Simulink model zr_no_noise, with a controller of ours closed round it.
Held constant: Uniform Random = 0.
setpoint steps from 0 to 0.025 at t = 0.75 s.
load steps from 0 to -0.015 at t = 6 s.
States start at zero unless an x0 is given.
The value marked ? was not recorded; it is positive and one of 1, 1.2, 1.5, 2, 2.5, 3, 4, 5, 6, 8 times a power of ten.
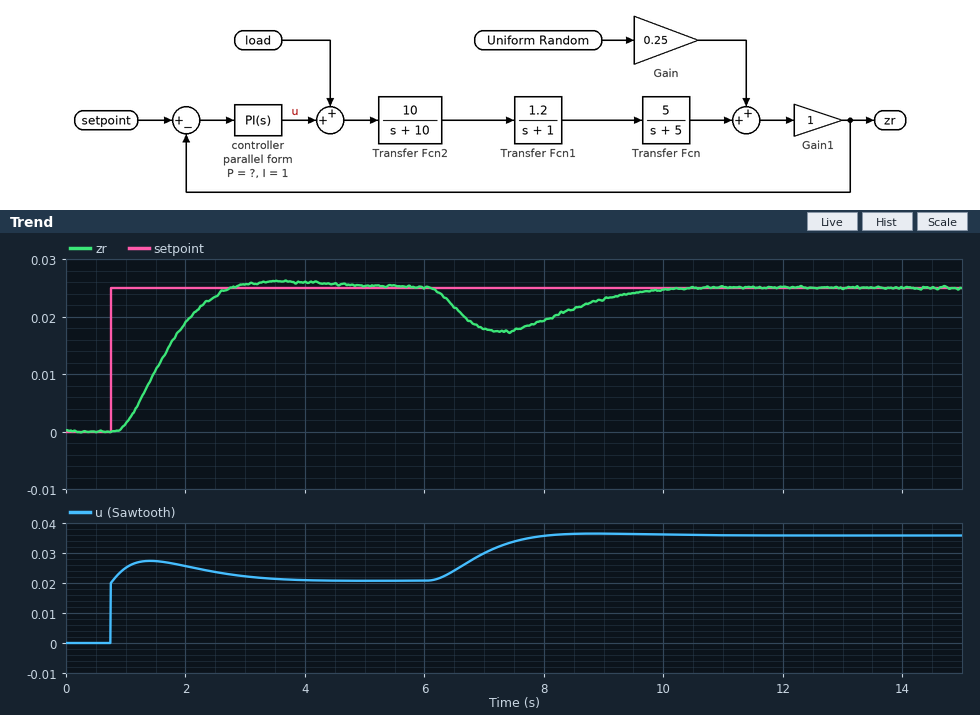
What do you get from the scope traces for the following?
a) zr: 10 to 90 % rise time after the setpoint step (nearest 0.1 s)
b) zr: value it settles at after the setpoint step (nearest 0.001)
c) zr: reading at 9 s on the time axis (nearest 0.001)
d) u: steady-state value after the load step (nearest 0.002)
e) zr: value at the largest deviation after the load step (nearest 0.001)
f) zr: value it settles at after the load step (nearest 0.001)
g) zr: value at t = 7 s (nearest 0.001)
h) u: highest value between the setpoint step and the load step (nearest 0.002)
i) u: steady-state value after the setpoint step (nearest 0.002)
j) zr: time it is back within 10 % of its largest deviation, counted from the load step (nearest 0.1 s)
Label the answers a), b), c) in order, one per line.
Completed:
a) 1.3 s
b) 0.025
c) 0.023
d) 0.036
e) 0.017
f) 0.025
g) 0.018
h) 0.028
i) 0.020
j) 3.6 s
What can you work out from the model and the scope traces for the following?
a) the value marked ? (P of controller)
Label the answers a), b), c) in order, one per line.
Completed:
a) 0.8
